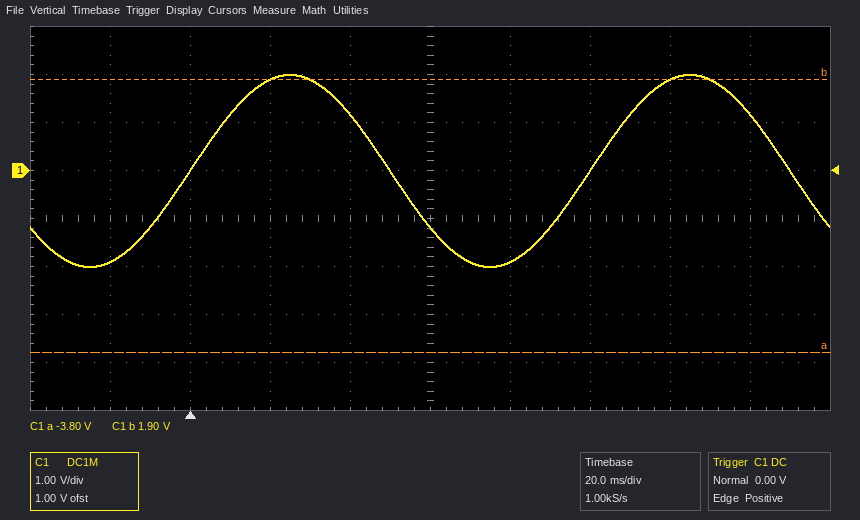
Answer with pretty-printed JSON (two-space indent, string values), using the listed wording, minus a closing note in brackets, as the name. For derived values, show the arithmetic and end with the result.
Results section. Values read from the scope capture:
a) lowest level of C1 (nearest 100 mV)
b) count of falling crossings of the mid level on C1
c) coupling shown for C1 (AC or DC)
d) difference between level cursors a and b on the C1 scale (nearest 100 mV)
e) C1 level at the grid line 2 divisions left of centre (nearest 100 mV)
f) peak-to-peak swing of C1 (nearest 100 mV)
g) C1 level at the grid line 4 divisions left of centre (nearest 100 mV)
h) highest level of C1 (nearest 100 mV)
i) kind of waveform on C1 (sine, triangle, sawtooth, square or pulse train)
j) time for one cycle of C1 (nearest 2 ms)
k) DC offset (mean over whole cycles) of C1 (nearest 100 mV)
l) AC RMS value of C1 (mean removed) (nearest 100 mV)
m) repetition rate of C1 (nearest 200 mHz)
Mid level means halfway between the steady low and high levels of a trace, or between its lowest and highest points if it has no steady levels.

{
  "lowest level of C1": "-2.0 V",
  "count of falling crossings of the mid level on C1": "2",
  "coupling shown for C1": "DC",
  "difference between level cursors a and b on the C1 scale": "5.7 V",
  "C1 level at the grid line 2 divisions left of centre": "1.9 V",
  "peak-to-peak swing of C1": "2.0 V − (-2.0 V) = 4.0 V",
  "C1 level at the grid line 4 divisions left of centre": "-1.9 V",
  "highest level of C1": "2.0 V",
  "kind of waveform on C1": "sine",
  "time for one cycle of C1": "100 ms",
  "DC offset (mean over whole cycles) of C1": "(2.0 V + (-2.0 V)) / 2 ≈ 0.0 V",
  "AC RMS value of C1 (mean removed)": "4.0 V / (2√2) ≈ 1.4 V",
  "repetition rate of C1": "1 / 100 ms ≈ 10.0 Hz"
}
